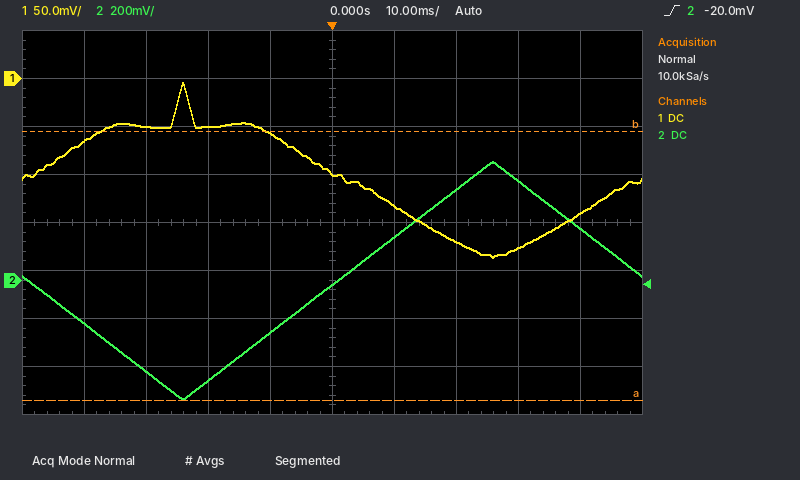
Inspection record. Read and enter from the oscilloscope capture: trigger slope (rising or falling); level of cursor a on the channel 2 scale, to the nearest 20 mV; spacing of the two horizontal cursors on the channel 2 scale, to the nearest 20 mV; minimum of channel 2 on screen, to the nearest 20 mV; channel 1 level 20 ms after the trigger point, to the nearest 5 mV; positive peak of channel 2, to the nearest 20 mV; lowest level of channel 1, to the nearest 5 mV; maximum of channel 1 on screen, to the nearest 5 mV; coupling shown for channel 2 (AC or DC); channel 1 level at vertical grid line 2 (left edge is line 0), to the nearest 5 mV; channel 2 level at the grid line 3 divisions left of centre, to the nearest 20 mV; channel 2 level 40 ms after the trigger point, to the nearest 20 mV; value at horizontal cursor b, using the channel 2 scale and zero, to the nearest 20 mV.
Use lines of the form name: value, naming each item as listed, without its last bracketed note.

trigger slope: rising
level of cursor a on the channel 2 scale, to the nearest 20 mV: -500 mV
spacing of the two horizontal cursors on the channel 2 scale, to the nearest 20 mV: 1.12 V
minimum of channel 2 on screen, to the nearest 20 mV: -500 mV
channel 1 level 20 ms after the trigger point, to the nearest 5 mV: -170 mV
positive peak of channel 2, to the nearest 20 mV: 500 mV
lowest level of channel 1, to the nearest 5 mV: -185 mV
maximum of channel 1 on screen, to the nearest 5 mV: -5 mV
coupling shown for channel 2: DC
channel 1 level at vertical grid line 2 (left edge is line 0), to the nearest 5 mV: -50 mV
channel 2 level at the grid line 3 divisions left of centre, to the nearest 20 mV: -380 mV
channel 2 level 40 ms after the trigger point, to the nearest 20 mV: 220 mV
value at horizontal cursor b, using the channel 2 scale and zero, to the nearest 20 mV: 620 mV
